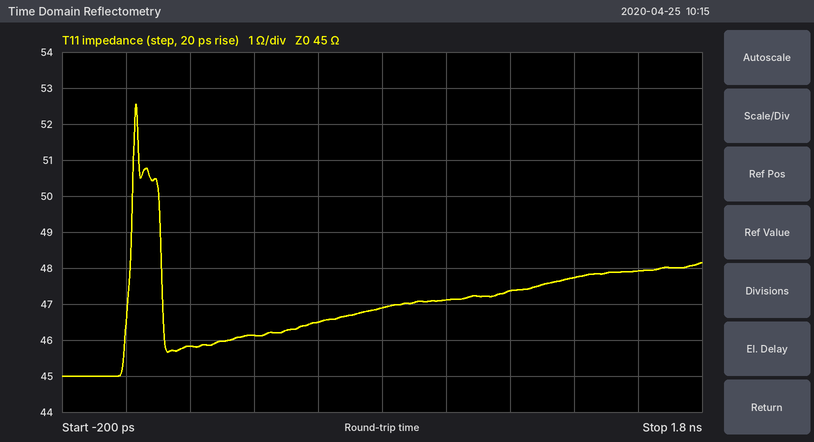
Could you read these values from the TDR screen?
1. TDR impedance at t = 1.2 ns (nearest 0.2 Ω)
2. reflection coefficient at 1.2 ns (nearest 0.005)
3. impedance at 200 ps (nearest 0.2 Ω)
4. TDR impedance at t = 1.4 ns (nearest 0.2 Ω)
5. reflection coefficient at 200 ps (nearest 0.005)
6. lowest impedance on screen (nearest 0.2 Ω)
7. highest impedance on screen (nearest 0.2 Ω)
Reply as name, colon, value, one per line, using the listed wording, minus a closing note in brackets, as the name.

TDR impedance at t = 1.2 ns: 47.4 Ω
reflection coefficient at 1.2 ns: +0.025
impedance at 200 ps: 45.8 Ω
TDR impedance at t = 1.4 ns: 47.8 Ω
reflection coefficient at 200 ps: +0.010
lowest impedance on screen: 45.0 Ω
highest impedance on screen: 52.6 Ω
